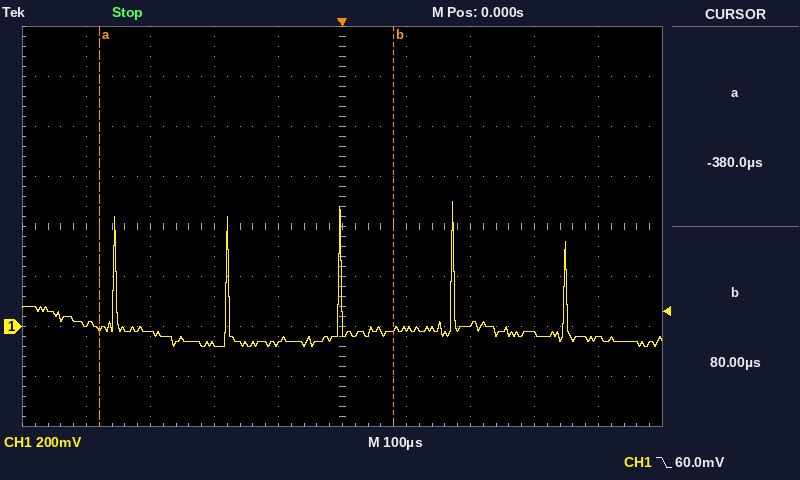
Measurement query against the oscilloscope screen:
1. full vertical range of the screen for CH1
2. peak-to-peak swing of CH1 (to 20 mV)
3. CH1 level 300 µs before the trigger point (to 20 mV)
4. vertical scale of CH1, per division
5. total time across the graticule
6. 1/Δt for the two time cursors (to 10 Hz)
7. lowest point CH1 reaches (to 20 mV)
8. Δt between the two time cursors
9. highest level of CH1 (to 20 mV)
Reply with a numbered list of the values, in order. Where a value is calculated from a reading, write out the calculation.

1. 1.6 V
2. 500 mV − (-80 mV) = 580 mV
3. -20 mV
4. 200 mV
5. 1 ms
6. 1 / 460 µs ≈ 2.17 kHz
7. -80 mV
8. 80 µs − (-380 µs) = 460 µs
9. 500 mV
